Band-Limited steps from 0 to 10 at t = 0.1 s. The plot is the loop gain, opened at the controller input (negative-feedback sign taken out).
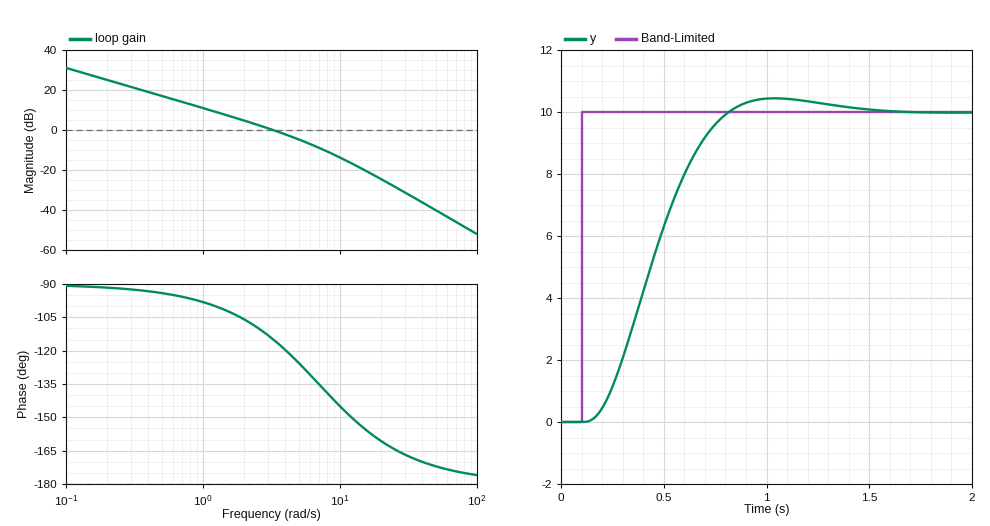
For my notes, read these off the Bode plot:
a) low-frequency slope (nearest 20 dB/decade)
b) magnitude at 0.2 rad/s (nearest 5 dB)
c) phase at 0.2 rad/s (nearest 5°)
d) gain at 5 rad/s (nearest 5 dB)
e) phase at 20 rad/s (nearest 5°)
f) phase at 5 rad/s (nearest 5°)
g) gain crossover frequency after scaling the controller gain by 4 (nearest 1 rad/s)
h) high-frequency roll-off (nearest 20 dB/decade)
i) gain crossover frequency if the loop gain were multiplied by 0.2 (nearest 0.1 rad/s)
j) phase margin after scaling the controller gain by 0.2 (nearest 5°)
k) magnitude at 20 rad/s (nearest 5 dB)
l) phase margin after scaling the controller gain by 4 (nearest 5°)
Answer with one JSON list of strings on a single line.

["-20 dB/decade", "25 dB", "-90°", "-5 dB", "-160°", "-125°", "9 rad/s", "-40 dB/decade", "0.7 rad/s", "85°", "-25 dB", "40°"]
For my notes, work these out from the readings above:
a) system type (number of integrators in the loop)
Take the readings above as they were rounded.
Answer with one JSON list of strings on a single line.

["1"]
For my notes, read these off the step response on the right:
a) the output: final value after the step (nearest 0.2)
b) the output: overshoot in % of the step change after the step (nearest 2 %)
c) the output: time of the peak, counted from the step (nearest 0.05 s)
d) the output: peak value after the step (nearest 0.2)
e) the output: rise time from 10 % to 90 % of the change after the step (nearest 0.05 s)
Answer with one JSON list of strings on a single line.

["10.0", "4 %", "0.95 s", "10.4", "0.45 s"]
